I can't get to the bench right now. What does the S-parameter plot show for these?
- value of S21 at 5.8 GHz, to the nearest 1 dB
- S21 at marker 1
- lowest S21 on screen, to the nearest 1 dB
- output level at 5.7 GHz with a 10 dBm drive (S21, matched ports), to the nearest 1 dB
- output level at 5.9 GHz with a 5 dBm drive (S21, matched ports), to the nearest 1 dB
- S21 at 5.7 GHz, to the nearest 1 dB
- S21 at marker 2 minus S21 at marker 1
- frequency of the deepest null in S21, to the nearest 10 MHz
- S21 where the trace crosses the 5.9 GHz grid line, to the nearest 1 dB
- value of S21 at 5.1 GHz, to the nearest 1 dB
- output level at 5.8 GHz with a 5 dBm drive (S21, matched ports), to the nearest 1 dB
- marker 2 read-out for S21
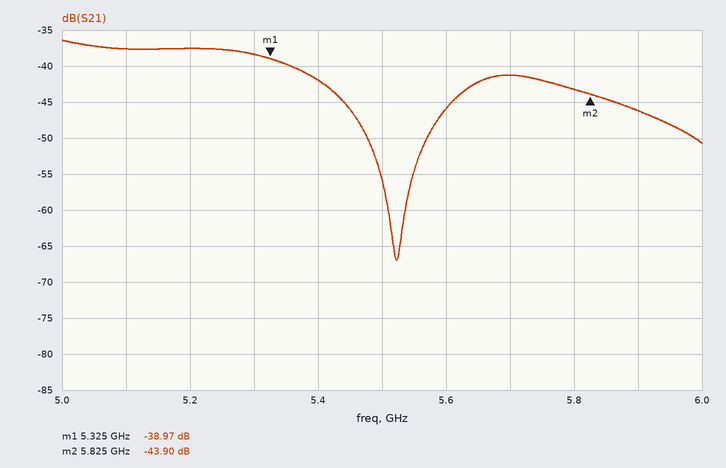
-43 dB
-38.97 dB
-67 dB
-31 dBm
-41 dBm
-41 dB
-4.93 dB
5.52 GHz
-46 dB
-38 dB
-38 dBm
-43.90 dB
